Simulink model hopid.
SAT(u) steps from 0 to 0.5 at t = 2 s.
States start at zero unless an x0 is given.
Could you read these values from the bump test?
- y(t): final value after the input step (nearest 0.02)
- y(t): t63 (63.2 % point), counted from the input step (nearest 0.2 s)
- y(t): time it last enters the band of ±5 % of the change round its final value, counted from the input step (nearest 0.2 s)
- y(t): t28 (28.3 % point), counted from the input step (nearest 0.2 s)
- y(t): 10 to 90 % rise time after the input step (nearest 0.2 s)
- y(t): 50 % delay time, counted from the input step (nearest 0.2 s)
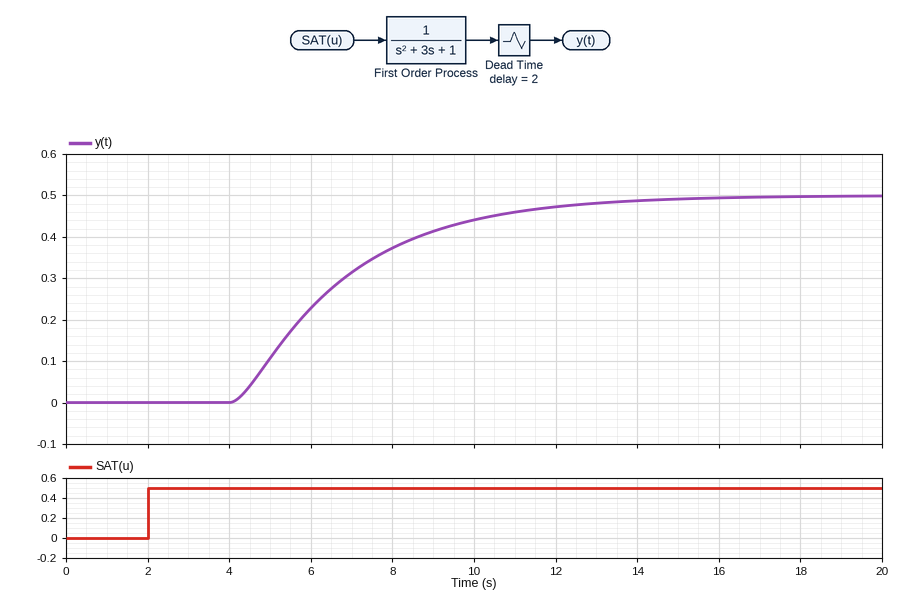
0.50
5.0 s
10.2 s
3.2 s
5.8 s
4.2 s
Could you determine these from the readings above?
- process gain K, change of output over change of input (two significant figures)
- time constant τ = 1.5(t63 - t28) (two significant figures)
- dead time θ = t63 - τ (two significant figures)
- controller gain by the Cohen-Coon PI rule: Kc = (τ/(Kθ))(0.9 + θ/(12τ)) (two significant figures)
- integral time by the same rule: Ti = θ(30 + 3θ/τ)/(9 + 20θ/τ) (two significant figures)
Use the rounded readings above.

1.0
2.7 s
2.3 s
1.1
2.9 s
